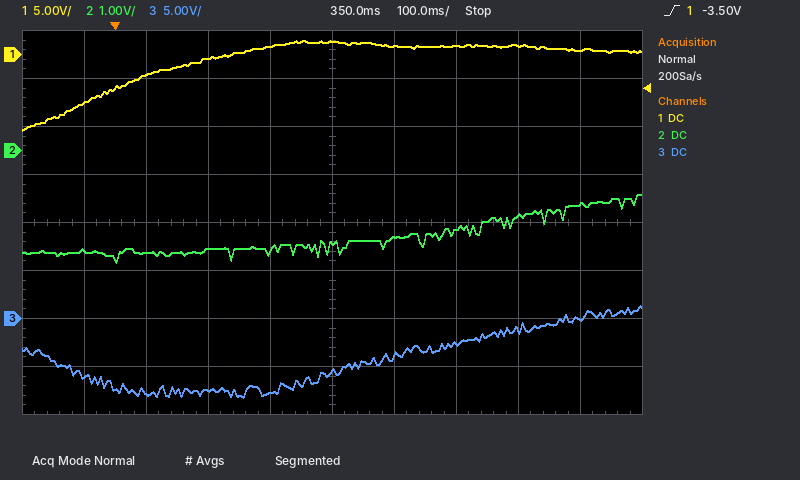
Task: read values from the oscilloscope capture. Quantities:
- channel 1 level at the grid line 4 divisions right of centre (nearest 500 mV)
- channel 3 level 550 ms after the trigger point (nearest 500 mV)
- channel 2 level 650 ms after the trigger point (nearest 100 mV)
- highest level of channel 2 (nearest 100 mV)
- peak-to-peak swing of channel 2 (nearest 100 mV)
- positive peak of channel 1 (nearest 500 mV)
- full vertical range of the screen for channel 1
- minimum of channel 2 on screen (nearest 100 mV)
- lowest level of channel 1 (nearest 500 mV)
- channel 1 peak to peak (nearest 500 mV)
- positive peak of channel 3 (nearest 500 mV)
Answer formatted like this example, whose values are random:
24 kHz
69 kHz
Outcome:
500 mV
-2.5 V
-1.4 V
-900 mV
1.4 V
1.5 V
40 V
-2.3 V
-8.0 V
9.5 V
1.5 V
